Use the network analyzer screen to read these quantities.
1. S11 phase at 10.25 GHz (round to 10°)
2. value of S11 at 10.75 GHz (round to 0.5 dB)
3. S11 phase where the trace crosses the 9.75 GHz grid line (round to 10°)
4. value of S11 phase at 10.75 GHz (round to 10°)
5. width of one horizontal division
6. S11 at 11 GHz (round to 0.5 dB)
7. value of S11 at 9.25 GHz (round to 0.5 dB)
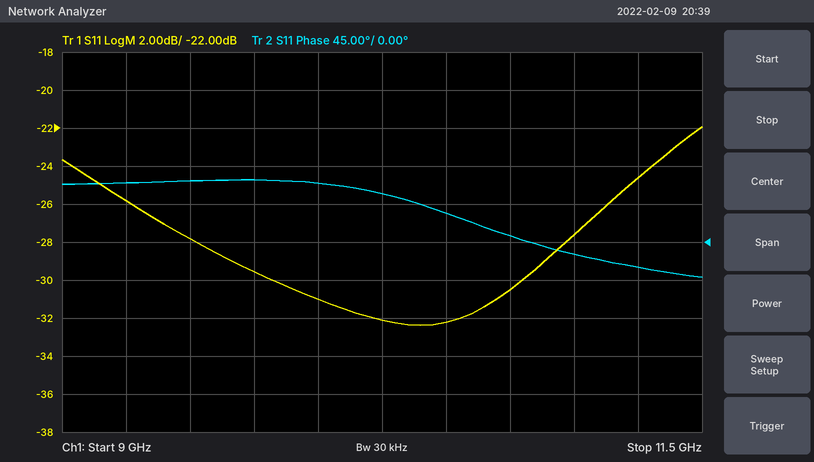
60°
-30.5 dB
70°
10°
250 MHz
-27.5 dB
-26.0 dB
